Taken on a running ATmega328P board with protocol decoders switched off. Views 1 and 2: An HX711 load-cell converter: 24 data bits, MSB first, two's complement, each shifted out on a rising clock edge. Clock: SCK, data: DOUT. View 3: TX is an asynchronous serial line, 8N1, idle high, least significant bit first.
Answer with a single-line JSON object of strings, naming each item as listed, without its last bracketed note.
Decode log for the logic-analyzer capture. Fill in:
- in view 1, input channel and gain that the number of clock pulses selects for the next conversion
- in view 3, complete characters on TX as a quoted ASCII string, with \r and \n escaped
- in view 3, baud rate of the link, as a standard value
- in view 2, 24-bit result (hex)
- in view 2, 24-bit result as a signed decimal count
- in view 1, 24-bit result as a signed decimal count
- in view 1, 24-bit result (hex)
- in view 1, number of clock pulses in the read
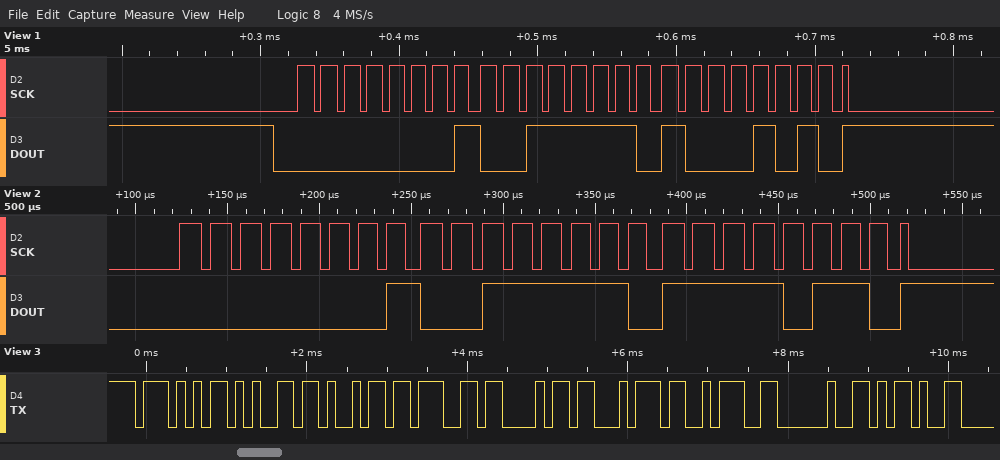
{"in view 1, input channel and gain that the number of clock pulses selects for the next conversion": "channel A, gain 128", "in view 3, complete characters on TX as a quoted ASCII string, with \\r and \\n escaped": "\"Weight: -\"", "in view 3, baud rate of the link, as a standard value": "9600 baud", "in view 2, 24-bit result": "0x013EF6", "in view 2, 24-bit result as a signed decimal count": "81654", "in view 1, 24-bit result as a signed decimal count": "81546", "in view 1, 24-bit result": "0x013E8A", "in view 1, number of clock pulses in the read": "25"}
